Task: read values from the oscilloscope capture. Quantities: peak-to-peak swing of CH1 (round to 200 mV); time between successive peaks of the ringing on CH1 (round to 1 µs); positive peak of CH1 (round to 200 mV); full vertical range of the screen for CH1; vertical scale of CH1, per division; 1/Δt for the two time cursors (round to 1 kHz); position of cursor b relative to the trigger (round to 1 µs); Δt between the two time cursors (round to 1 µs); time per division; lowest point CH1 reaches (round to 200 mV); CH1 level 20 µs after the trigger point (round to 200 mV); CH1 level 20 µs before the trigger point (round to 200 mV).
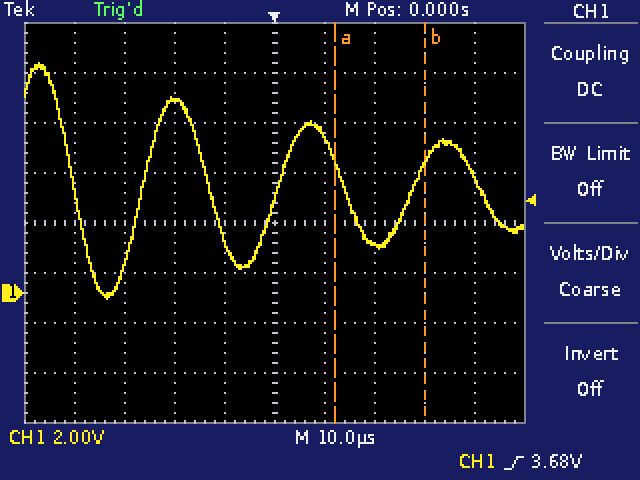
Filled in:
9.4 V
27 µs
9.2 V
16 V
2 V
56 kHz
+30 µs
18 µs
10 µs
-200 mV
2.0 V
7.8 V
